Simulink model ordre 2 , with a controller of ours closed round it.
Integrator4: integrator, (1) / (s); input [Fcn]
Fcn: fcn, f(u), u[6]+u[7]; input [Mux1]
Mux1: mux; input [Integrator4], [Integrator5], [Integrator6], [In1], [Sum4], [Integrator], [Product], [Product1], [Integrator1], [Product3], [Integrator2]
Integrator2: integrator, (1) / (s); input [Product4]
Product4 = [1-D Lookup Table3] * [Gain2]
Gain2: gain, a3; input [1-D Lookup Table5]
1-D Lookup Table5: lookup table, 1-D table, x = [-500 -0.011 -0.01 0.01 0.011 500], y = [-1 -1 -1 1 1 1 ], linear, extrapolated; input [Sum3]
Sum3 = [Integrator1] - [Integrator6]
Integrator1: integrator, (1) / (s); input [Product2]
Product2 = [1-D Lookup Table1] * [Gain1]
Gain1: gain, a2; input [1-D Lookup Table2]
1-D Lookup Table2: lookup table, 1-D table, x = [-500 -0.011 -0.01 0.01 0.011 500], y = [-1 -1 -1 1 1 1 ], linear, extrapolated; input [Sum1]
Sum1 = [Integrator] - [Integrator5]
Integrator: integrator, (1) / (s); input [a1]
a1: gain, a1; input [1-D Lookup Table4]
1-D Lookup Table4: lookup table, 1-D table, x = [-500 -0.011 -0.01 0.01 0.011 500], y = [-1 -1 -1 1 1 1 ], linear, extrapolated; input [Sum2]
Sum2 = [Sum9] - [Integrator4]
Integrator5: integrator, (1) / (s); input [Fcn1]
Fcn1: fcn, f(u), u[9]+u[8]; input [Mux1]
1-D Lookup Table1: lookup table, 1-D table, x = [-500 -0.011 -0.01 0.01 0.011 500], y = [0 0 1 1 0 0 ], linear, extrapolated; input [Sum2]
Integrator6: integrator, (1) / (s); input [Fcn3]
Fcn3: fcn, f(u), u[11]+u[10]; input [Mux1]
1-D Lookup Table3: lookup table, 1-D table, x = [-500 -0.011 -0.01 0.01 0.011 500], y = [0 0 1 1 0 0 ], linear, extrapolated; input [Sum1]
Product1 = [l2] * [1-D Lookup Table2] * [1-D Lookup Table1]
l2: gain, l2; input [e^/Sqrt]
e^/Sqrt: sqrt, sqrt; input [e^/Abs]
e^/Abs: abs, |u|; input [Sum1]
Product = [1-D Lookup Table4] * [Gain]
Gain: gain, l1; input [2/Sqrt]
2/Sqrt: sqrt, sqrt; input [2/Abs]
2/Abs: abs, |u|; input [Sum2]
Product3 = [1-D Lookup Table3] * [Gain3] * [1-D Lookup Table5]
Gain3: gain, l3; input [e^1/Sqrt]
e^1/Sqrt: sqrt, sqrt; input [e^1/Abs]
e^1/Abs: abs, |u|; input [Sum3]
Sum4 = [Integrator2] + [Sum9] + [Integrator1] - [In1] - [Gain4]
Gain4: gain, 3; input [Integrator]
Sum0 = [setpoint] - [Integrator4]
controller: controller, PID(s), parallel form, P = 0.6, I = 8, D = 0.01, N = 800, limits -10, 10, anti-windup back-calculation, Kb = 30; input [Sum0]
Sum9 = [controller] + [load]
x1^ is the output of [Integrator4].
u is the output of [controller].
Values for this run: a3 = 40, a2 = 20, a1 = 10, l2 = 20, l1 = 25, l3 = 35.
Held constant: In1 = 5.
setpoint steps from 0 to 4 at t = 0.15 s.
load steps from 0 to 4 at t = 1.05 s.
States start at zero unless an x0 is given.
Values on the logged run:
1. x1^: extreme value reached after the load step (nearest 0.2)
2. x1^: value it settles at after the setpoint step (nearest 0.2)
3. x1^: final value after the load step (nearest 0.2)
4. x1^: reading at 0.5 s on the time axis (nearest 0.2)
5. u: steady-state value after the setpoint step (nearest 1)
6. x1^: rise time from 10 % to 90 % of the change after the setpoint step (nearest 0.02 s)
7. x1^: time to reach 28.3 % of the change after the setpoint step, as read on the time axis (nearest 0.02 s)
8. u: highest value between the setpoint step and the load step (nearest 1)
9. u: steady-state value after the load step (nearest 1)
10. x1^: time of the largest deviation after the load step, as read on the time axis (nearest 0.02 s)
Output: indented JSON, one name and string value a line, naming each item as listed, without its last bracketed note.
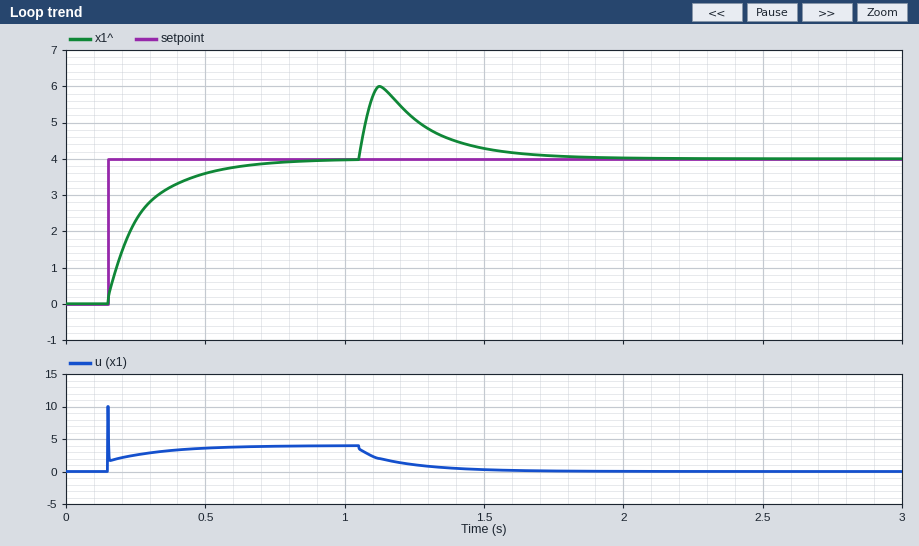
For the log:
{
  "x1^: extreme value reached after the load step": "6.0",
  "x1^: value it settles at after the setpoint step": "4.0",
  "x1^: final value after the load step": "4.0",
  "x1^: reading at 0.5 s on the time axis": "3.6",
  "u: steady-state value after the setpoint step": "4",
  "x1^: rise time from 10 % to 90 % of the change after the setpoint step": "0.34 s",
  "x1^: time to reach 28.3 % of the change after the setpoint step, as read on the time axis": "0.18 s",
  "u: highest value between the setpoint step and the load step": "10",
  "u: steady-state value after the load step": "0",
  "x1^: time of the largest deviation after the load step, as read on the time axis": "1.12 s"
}
